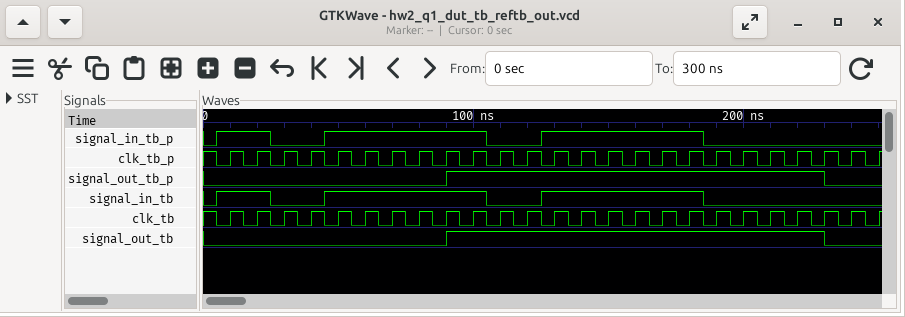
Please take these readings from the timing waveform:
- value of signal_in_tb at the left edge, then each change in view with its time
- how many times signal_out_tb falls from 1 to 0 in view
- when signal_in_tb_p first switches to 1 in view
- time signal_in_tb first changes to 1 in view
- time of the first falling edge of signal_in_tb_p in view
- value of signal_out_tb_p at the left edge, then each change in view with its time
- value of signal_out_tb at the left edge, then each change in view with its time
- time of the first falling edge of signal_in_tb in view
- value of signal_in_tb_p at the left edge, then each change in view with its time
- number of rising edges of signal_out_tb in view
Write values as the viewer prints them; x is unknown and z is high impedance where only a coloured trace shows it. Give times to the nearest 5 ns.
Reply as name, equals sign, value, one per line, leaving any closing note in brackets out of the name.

value of signal_in_tb at the left edge, then each change in view with its time = 0, 1 at 5 ns, 0 at 25 ns, 1 at 45 ns, 0 at 105 ns, 1 at 125 ns, 0 at 185 ns
how many times signal_out_tb falls from 1 to 0 in view = 1
when signal_in_tb_p first switches to 1 in view = 5 ns
time signal_in_tb first changes to 1 in view = 5 ns
time of the first falling edge of signal_in_tb_p in view = 25 ns
value of signal_out_tb_p at the left edge, then each change in view with its time = 0, 1 at 90 ns, 0 at 230 ns
value of signal_out_tb at the left edge, then each change in view with its time = 0, 1 at 90 ns, 0 at 230 ns
time of the first falling edge of signal_in_tb in view = 25 ns
value of signal_in_tb_p at the left edge, then each change in view with its time = 0, 1 at 5 ns, 0 at 25 ns, 1 at 45 ns, 0 at 105 ns, 1 at 125 ns, 0 at 185 ns
number of rising edges of signal_out_tb in view = 1
